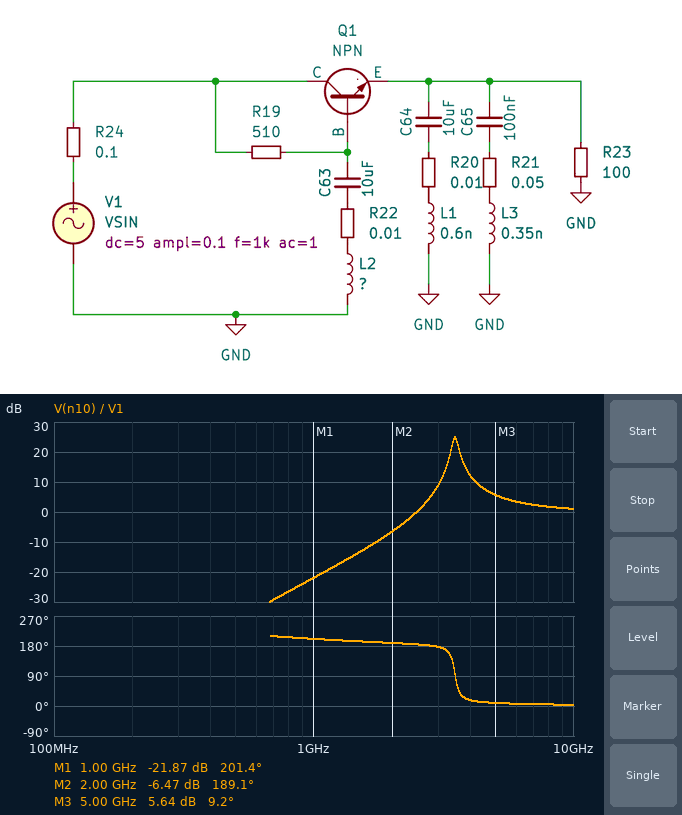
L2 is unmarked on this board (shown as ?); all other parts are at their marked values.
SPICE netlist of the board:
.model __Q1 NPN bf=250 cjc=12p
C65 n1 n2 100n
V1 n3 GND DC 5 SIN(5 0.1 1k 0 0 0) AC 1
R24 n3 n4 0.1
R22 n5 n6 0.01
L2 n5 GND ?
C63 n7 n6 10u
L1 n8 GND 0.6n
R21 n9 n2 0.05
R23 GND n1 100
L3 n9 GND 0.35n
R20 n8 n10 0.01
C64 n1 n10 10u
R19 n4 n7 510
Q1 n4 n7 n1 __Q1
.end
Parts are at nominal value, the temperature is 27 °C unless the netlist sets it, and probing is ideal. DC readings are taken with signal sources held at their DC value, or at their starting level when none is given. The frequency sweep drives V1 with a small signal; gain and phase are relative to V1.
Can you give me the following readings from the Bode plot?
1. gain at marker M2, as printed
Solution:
-6.47 dB
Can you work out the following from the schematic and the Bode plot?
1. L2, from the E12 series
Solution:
180 pH
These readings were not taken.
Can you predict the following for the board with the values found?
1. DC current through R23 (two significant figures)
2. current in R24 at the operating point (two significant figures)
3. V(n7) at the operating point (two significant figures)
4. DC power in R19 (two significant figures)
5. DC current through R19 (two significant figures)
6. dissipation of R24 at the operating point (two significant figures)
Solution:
40 mA
40 mA
4.9 V
13 µW
160 µA
160 µW
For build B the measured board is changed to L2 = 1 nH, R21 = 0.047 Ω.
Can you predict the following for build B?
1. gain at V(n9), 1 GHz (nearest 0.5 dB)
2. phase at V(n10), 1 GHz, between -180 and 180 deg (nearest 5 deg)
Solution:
-2.5 dB
-165 deg
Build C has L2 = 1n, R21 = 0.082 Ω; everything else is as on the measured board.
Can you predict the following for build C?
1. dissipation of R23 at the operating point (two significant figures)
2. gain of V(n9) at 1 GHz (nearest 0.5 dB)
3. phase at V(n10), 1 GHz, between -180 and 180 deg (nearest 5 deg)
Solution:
160 mW
-2.5 dB
-165 deg
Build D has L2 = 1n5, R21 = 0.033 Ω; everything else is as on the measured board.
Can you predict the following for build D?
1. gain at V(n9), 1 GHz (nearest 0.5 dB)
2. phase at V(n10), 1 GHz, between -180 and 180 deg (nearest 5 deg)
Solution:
5.5 dB
-170 deg
